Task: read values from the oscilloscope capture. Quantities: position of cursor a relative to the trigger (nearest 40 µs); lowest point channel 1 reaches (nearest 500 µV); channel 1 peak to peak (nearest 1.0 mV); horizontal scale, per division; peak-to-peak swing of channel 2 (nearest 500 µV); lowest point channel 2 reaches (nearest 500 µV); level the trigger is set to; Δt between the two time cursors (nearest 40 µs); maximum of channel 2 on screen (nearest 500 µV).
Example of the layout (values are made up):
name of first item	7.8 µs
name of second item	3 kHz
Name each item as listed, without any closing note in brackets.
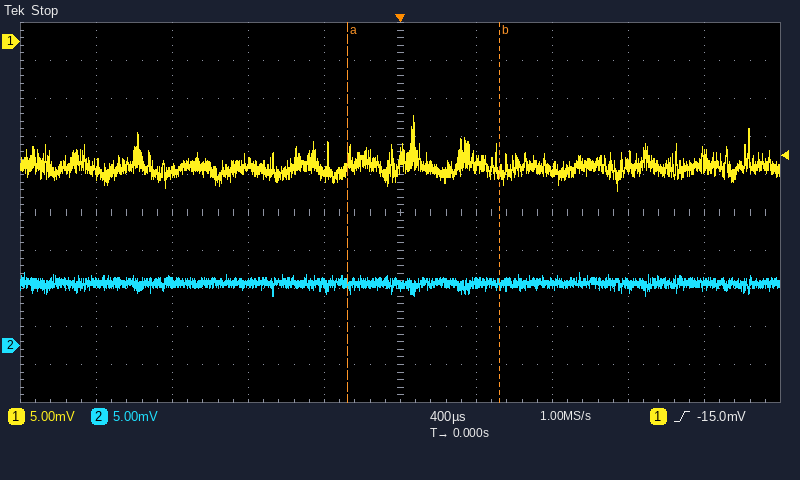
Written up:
position of cursor a relative to the trigger	-280 µs
lowest point channel 1 reaches	-19.5 mV
channel 1 peak to peak	10.0 mV
horizontal scale, per division	400 µs
peak-to-peak swing of channel 2	3.0 mV
lowest point channel 2 reaches	6.5 mV
level the trigger is set to	-15.0 mV
Δt between the two time cursors	800 µs
maximum of channel 2 on screen	9.5 mV
